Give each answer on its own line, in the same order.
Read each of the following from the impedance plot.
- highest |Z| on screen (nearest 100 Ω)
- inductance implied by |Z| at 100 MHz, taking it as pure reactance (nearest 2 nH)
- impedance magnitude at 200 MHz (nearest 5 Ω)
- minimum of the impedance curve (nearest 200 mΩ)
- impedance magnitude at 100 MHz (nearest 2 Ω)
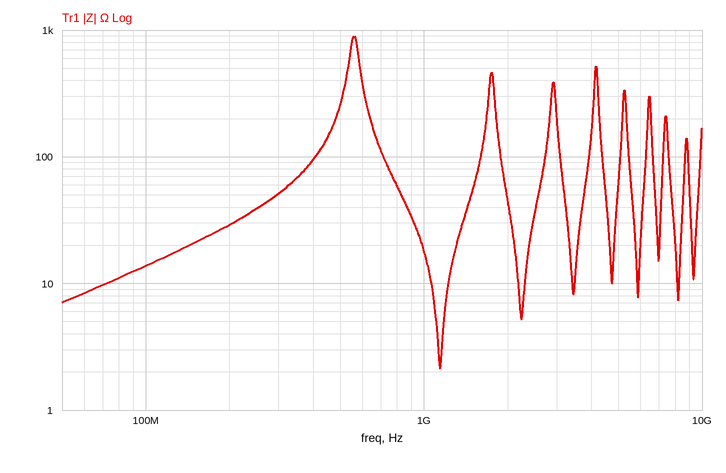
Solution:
900 Ω
22 nH
30 Ω
2.2 Ω
14 Ω
